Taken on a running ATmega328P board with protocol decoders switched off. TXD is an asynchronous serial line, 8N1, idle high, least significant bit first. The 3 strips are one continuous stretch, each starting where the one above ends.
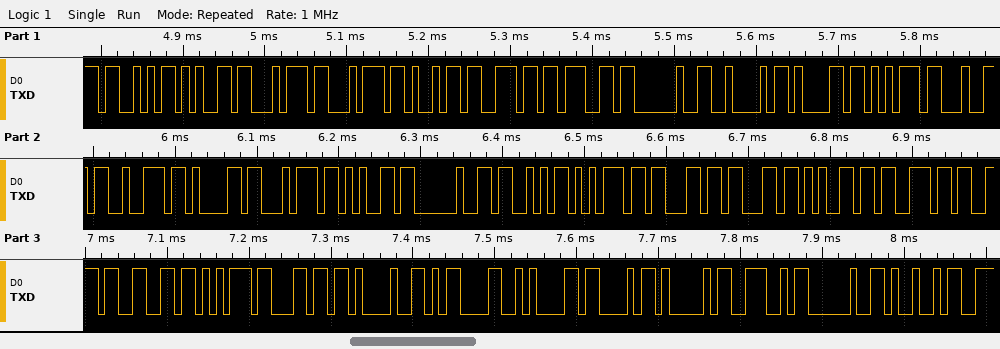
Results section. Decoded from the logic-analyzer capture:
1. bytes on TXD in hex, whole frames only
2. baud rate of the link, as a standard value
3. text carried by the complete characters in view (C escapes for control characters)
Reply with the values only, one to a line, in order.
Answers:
53 65 74 74 69 6E 67 20 42 61 75 64 72 61 74 65 20 53 75 63 63 65 73 73 66 75 6C 21 0D 0A 43 41 4E 20 49
115200 baud
"Setting Baudrate Successful!\r\nCAN I"
